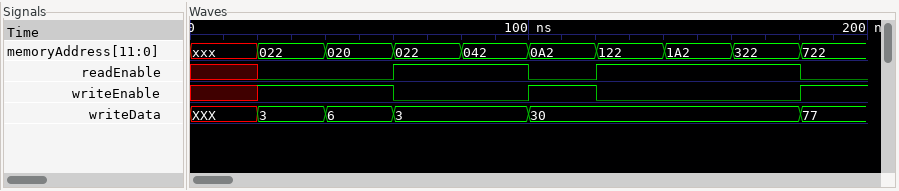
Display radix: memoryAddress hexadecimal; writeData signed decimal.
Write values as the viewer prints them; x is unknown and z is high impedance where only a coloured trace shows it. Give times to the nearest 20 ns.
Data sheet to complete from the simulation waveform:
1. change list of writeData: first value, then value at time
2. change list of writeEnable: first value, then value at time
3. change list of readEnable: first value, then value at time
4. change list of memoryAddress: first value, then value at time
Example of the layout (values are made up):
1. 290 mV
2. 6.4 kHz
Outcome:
1. XXX, 3 at 20 ns, 6 at 40 ns, 3 at 60 ns, 30 at 100 ns, 77 at 180 ns
2. x, 1 at 20 ns, 0 at 60 ns, 1 at 100 ns, 0 at 120 ns, 1 at 180 ns
3. x, 0 at 20 ns, 1 at 60 ns, 0 at 100 ns, 1 at 120 ns, 0 at 180 ns
4. xxx, 022 at 20 ns, 020 at 40 ns, 022 at 60 ns, 042 at 80 ns, 0A2 at 100 ns, 122 at 120 ns, 1A2 at 140 ns, 322 at 160 ns, 722 at 180 ns
